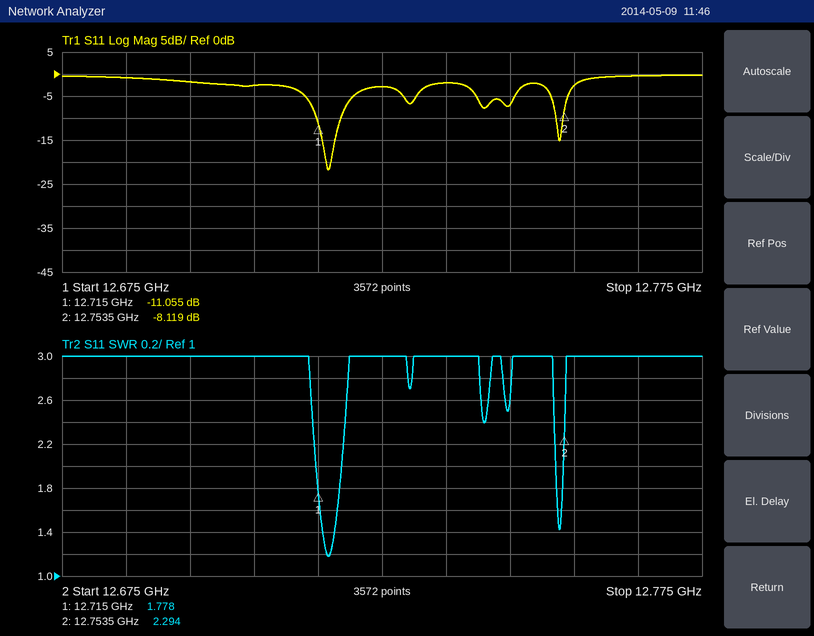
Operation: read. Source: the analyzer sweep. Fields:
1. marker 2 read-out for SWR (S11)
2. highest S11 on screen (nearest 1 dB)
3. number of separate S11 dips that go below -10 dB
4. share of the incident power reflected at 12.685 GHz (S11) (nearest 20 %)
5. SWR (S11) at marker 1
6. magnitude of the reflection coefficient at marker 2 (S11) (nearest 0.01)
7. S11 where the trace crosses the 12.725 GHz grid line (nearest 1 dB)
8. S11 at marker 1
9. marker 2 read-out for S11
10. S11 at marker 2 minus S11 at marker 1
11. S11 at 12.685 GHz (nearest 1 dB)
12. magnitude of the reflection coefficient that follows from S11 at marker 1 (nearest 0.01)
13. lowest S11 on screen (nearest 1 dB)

2.294
0 dB
2
80 %
1.778
0.39
-3 dB
-11.055 dB
-8.119 dB
2.936 dB
-1 dB
0.28
-22 dB
